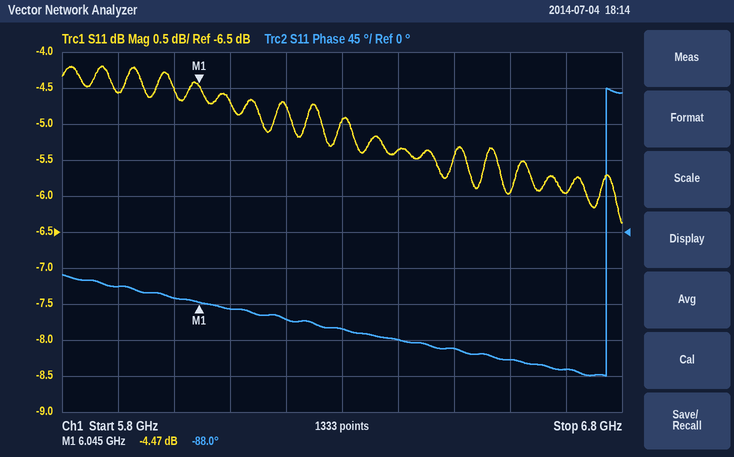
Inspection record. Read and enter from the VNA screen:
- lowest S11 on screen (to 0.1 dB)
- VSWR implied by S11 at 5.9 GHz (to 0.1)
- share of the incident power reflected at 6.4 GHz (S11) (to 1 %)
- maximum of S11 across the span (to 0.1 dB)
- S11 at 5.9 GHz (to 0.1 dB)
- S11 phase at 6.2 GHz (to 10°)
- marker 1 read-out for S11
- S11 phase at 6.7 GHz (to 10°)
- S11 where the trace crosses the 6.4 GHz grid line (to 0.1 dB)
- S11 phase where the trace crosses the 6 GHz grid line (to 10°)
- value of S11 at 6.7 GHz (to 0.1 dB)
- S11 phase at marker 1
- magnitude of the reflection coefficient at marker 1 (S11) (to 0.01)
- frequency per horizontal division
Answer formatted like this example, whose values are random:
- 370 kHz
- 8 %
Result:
- -6.4 dB
- 3.9
- 29 %
- -4.2 dB
- -4.6 dB
- -110°
- -4.47 dB
- -170°
- -5.4 dB
- -80°
- -6.0 dB
- -88.0°
- 0.60
- 100 MHz
